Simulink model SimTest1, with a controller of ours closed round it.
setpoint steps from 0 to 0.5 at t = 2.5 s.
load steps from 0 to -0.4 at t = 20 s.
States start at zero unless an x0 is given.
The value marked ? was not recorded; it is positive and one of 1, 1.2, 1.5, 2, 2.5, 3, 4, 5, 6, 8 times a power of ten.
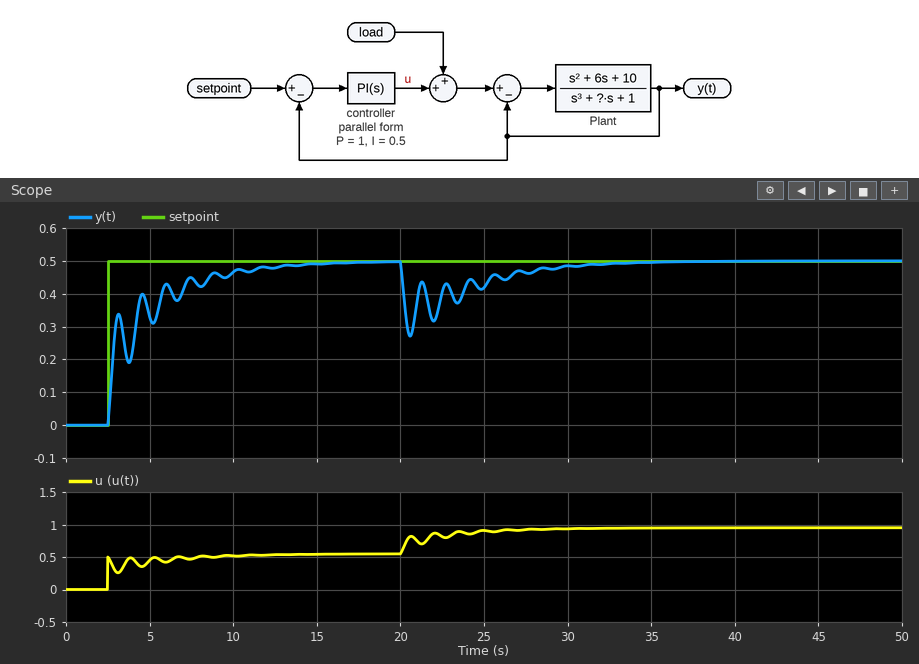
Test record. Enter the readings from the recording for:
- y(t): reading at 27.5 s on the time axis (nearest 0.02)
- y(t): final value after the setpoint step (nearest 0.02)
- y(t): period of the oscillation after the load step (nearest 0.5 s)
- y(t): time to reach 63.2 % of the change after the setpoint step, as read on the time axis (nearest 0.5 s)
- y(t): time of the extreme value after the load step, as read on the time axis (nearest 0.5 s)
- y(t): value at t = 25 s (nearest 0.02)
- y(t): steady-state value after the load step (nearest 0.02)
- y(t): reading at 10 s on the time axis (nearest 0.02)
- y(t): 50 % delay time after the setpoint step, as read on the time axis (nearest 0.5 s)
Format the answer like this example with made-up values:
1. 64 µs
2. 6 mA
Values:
1. 0.46
2. 0.50
3. 1.5 s
4. 3.0 s
5. 20.5 s
6. 0.42
7. 0.50
8. 0.46
9. 3.0 s
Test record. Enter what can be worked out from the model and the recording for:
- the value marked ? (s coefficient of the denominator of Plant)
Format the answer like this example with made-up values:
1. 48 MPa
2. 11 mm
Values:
1. 8
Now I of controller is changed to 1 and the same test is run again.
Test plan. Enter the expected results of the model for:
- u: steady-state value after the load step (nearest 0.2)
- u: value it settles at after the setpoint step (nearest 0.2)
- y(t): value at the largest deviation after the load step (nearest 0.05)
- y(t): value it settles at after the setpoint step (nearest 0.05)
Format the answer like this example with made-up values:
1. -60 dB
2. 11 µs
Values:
1. 1.0
2. 0.6
3. 0.30
4. 0.50
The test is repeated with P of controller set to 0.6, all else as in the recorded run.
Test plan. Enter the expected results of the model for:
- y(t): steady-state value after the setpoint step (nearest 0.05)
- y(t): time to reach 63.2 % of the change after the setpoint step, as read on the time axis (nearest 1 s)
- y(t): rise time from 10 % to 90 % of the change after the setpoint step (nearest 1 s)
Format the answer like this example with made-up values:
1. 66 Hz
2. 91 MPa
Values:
1. 0.50
2. 4 s
3. 5 s
